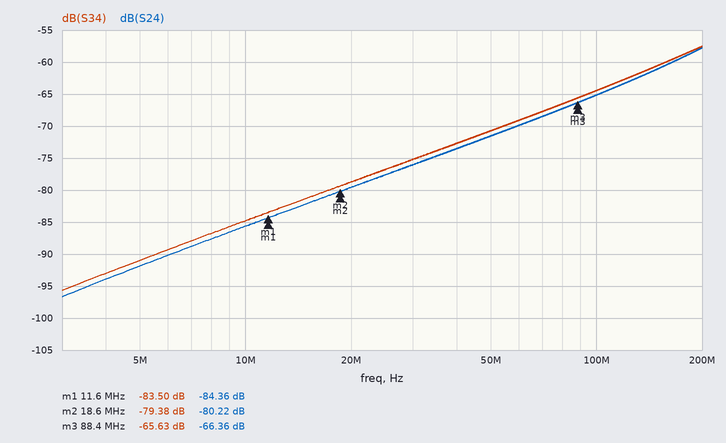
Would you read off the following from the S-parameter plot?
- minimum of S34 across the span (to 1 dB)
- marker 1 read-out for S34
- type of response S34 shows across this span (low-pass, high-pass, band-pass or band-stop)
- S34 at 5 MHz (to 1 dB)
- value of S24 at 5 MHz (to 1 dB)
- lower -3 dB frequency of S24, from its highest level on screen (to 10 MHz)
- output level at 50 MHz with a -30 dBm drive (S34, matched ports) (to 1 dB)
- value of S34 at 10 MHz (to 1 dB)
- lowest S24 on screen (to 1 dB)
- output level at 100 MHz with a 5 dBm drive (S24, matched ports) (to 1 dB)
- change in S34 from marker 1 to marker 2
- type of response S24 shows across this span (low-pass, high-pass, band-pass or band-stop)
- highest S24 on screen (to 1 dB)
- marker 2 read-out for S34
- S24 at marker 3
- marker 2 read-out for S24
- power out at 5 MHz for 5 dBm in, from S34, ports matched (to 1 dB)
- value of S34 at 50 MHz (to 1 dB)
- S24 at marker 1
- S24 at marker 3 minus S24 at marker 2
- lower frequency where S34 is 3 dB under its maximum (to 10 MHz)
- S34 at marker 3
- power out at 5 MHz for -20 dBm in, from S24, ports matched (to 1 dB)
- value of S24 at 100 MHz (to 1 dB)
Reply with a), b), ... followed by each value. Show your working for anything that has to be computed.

a) -96 dB
b) -83.50 dB
c) high-pass
d) -91 dB
e) -92 dB
f) 150 MHz
g) -30 dBm + (-71 dB) = -101 dBm
h) -85 dB
i) -97 dB
j) 5 dBm + (-65 dB) = -60 dBm
k) -79.38 − (-83.5) = 4.12 dB
l) high-pass
m) -58 dB
n) -79.38 dB
o) -66.36 dB
p) -80.22 dB
q) 5 dBm + (-91 dB) = -86 dBm
r) -71 dB
s) -84.36 dB
t) -66.36 − (-80.22) = 13.86 dB
u) 150 MHz
v) -65.63 dB
w) -20 dBm + (-92 dB) = -112 dBm
x) -65 dB
